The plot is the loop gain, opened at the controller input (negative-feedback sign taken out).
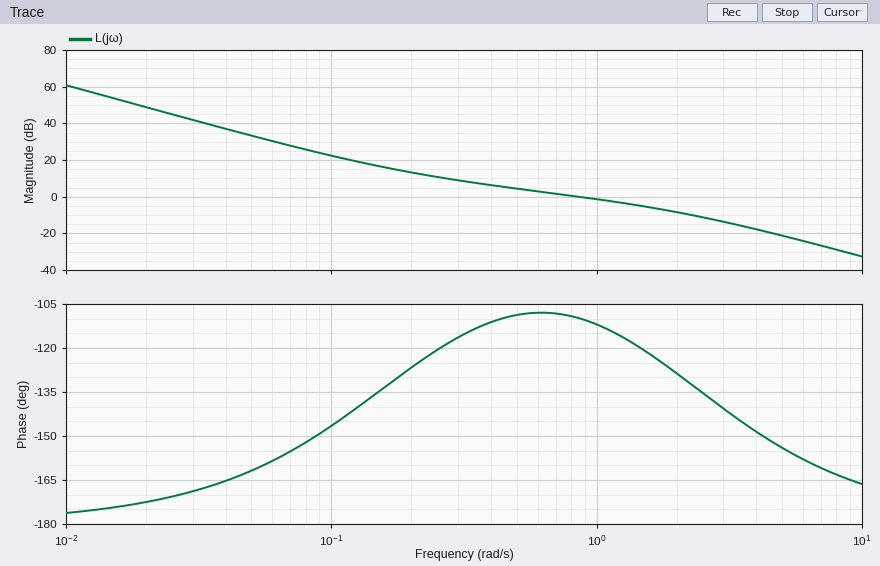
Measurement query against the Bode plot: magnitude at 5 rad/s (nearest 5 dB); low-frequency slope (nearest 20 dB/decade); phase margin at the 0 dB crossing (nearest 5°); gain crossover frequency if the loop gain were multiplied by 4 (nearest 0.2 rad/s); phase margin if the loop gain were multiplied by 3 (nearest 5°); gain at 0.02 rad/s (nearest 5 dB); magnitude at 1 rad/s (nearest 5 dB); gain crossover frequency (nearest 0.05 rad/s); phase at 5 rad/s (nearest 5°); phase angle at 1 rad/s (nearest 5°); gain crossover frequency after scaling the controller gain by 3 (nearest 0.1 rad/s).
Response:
-20 dB
-40 dB/decade
70°
2.6 rad/s
50°
50 dB
0 dB
0.85 rad/s
-155°
-110°
2.2 rad/s
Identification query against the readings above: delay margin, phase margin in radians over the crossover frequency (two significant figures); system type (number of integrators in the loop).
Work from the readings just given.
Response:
1.4 s
2
